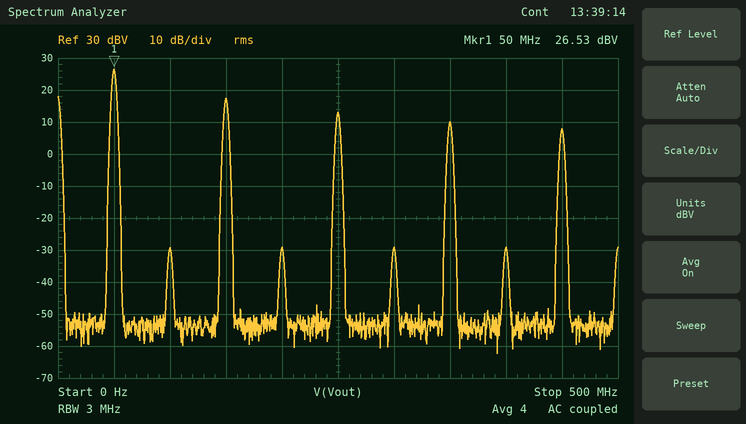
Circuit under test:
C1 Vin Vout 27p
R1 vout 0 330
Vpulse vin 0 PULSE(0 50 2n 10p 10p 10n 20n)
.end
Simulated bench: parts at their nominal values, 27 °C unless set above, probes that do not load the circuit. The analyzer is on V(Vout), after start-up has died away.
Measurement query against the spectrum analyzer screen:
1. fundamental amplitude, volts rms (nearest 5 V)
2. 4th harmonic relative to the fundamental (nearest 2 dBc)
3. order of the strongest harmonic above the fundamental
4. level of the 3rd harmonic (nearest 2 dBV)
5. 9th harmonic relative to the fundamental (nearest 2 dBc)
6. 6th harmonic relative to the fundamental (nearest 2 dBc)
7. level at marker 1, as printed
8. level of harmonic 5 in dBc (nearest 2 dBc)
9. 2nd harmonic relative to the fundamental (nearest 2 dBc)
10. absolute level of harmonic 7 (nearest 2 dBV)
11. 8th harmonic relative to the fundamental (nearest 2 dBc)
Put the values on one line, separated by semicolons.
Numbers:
20 V; -56 dBc; 3; 18 dBV; -18 dBc; -56 dBc; 26.53 dBV; -14 dBc; -56 dBc; 10 dBV; -56 dBc
